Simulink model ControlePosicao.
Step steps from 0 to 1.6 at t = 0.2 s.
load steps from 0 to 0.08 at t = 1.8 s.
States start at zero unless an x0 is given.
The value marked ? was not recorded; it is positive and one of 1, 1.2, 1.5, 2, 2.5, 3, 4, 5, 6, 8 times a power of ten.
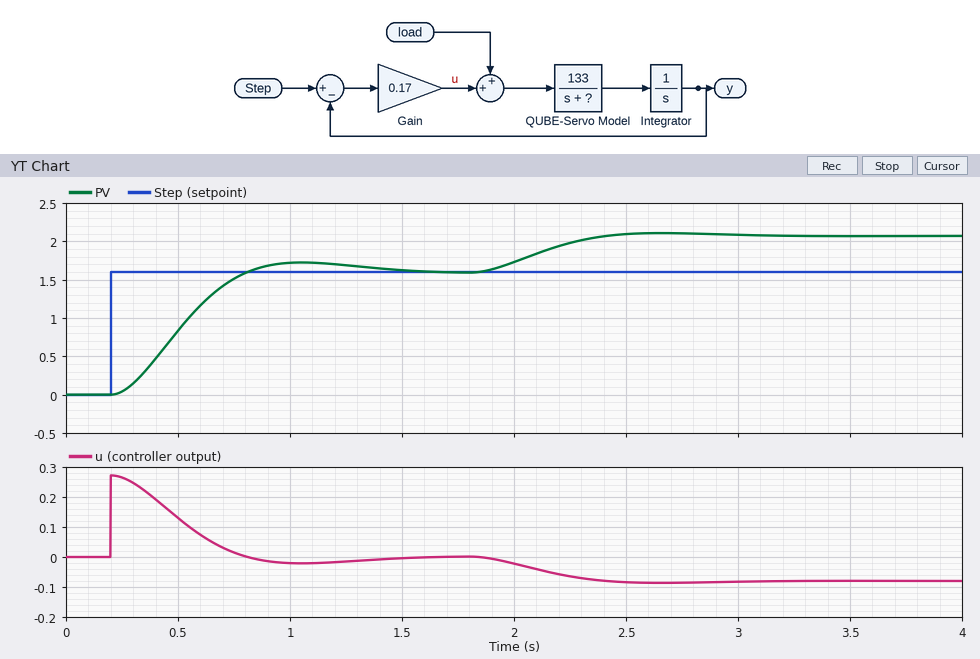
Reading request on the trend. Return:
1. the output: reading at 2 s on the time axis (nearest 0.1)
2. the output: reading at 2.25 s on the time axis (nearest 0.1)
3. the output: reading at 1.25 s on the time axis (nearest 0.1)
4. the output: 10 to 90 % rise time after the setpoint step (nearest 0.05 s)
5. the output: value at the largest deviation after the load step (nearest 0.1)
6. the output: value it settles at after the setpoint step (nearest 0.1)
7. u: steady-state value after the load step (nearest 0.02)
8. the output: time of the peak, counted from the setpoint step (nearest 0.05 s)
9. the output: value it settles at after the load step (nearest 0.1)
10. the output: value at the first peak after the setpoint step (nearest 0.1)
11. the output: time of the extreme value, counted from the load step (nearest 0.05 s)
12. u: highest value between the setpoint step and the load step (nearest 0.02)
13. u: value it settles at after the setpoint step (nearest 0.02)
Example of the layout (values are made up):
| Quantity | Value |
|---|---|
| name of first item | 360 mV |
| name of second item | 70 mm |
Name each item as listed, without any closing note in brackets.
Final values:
| Quantity | Value |
|---|---|
| the output: reading at 2 s on the time axis | 1.7 |
| the output: reading at 2.25 s on the time axis | 2.0 |
| the output: reading at 1.25 s on the time axis | 1.7 |
| the output: 10 to 90 % rise time after the setpoint step | 0.40 s |
| the output: value at the largest deviation after the load step | 2.1 |
| the output: value it settles at after the setpoint step | 1.6 |
| u: steady-state value after the load step | -0.08 |
| the output: time of the peak, counted from the setpoint step | 0.85 s |
| the output: value it settles at after the load step | 2.1 |
| the output: value at the first peak after the setpoint step | 1.7 |
| the output: time of the extreme value, counted from the load step | 0.85 s |
| u: highest value between the setpoint step and the load step | 0.28 |
| u: value it settles at after the setpoint step | 0.00 |
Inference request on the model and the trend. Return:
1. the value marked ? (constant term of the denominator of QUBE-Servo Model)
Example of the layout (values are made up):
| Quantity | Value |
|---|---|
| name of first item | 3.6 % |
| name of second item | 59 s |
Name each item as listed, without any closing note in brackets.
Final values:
| Quantity | Value |
|---|---|
| the value marked ? | 6 |
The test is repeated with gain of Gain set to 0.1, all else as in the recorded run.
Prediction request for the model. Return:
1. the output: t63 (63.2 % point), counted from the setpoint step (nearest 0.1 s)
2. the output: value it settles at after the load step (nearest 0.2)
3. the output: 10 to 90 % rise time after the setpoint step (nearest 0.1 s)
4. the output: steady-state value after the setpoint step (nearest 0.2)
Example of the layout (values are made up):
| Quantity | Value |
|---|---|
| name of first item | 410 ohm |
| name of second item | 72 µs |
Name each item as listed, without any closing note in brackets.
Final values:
| Quantity | Value |
|---|---|
| the output: t63 (63.2 % point), counted from the setpoint step | 0.5 s |
| the output: value it settles at after the load step | 2.4 |
| the output: 10 to 90 % rise time after the setpoint step | 0.7 s |
| the output: steady-state value after the setpoint step | 1.6 |
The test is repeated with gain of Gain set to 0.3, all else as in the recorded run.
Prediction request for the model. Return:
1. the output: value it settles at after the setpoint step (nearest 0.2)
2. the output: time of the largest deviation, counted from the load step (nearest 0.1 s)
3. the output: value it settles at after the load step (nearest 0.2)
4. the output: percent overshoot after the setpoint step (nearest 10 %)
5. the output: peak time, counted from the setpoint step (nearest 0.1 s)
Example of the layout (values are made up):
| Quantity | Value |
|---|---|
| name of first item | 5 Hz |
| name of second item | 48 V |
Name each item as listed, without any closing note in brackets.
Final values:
| Quantity | Value |
|---|---|
| the output: value it settles at after the setpoint step | 1.6 |
| the output: time of the largest deviation, counted from the load step | 0.6 s |
| the output: value it settles at after the load step | 1.8 |
| the output: percent overshoot after the setpoint step | 20 % |
| the output: peak time, counted from the setpoint step | 0.6 s |
